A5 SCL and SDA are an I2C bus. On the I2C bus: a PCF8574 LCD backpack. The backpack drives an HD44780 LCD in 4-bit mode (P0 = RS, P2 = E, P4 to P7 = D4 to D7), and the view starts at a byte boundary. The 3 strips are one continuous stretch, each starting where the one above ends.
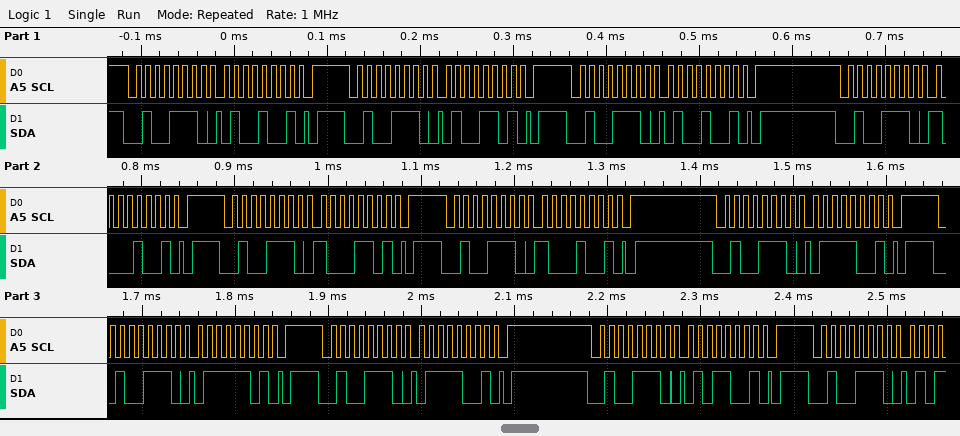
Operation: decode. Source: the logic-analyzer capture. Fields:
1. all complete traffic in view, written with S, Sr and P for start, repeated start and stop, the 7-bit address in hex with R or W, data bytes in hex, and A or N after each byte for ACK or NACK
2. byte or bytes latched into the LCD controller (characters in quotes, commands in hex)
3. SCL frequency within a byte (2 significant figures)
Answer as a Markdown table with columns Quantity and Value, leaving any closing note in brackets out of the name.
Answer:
| Quantity | Value |
|---|---|
| all complete traffic in view, written with S, Sr and P for start, repeated start and stop, the 7-bit address in hex with R or W, data bytes in hex, and A or N after each byte for ACK or NACK | S 27W A 49 A P S 27W A 4D A P S 27W A 49 A P S 27W A 89 A P S 27W A 8D A P S 27W A 89 A P S 27W A 79 A P S 27W A 7D A P S 27W A 79 A P S 27W A 59 A P S 27W A |
| byte or bytes latched into the LCD controller | 'H' |
| SCL frequency within a byte | 100 kHz |
